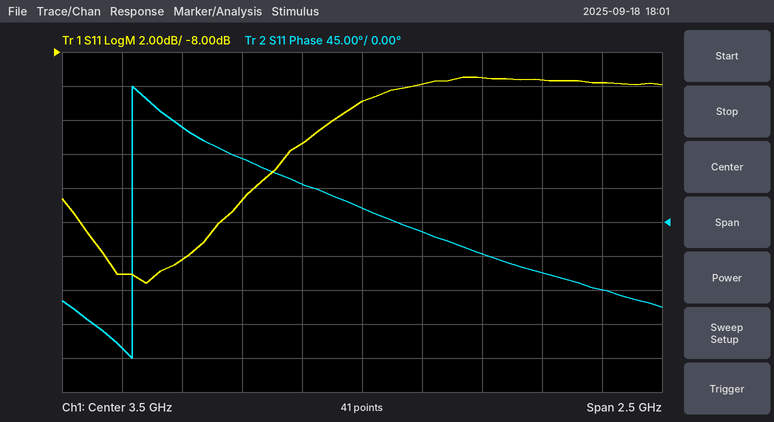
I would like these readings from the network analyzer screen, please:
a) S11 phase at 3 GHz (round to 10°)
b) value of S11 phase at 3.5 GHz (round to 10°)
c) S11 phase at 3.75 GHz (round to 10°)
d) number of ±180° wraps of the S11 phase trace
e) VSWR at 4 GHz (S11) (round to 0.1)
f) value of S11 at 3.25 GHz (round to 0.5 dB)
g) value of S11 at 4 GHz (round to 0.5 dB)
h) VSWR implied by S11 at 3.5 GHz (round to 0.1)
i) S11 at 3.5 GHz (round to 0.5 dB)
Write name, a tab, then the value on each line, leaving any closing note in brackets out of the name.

S11 phase at 3 GHz	80°
value of S11 phase at 3.5 GHz	20°
S11 phase at 3.75 GHz	-10°
number of ±180° wraps of the S11 phase trace	1
VSWR at 4 GHz (S11)	2.0
value of S11 at 3.25 GHz	-13.5 dB
value of S11 at 4 GHz	-9.5 dB
VSWR implied by S11 at 3.5 GHz	1.8
S11 at 3.5 GHz	-11.0 dB
